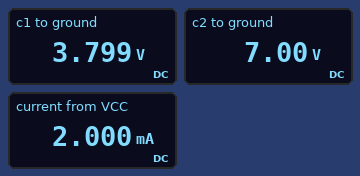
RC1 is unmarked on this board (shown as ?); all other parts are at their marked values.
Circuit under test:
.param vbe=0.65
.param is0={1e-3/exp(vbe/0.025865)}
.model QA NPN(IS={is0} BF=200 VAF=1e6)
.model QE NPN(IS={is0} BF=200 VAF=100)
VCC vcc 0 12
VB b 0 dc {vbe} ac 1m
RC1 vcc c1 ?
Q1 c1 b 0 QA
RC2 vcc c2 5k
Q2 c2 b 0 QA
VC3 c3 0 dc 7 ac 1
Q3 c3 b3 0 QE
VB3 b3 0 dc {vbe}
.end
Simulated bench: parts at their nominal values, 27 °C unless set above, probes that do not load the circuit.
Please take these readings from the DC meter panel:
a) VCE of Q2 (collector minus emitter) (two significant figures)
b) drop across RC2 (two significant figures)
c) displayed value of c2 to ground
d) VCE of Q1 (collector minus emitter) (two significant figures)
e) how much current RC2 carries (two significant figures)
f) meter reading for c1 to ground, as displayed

7.0 V
5.0 V
7.00 V
3.8 V
1.0 mA
3.799 V
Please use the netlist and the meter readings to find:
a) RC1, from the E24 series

8.2 kΩ
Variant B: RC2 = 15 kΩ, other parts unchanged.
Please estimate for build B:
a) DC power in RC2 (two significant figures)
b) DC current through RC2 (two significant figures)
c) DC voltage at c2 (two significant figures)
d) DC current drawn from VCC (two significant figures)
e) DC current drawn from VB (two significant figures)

9.5 mW
800 µA
59 mV
1.8 mA
110 µA
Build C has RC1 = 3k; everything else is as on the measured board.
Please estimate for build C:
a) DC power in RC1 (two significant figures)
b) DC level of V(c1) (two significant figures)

3.0 mW
9.0 V
